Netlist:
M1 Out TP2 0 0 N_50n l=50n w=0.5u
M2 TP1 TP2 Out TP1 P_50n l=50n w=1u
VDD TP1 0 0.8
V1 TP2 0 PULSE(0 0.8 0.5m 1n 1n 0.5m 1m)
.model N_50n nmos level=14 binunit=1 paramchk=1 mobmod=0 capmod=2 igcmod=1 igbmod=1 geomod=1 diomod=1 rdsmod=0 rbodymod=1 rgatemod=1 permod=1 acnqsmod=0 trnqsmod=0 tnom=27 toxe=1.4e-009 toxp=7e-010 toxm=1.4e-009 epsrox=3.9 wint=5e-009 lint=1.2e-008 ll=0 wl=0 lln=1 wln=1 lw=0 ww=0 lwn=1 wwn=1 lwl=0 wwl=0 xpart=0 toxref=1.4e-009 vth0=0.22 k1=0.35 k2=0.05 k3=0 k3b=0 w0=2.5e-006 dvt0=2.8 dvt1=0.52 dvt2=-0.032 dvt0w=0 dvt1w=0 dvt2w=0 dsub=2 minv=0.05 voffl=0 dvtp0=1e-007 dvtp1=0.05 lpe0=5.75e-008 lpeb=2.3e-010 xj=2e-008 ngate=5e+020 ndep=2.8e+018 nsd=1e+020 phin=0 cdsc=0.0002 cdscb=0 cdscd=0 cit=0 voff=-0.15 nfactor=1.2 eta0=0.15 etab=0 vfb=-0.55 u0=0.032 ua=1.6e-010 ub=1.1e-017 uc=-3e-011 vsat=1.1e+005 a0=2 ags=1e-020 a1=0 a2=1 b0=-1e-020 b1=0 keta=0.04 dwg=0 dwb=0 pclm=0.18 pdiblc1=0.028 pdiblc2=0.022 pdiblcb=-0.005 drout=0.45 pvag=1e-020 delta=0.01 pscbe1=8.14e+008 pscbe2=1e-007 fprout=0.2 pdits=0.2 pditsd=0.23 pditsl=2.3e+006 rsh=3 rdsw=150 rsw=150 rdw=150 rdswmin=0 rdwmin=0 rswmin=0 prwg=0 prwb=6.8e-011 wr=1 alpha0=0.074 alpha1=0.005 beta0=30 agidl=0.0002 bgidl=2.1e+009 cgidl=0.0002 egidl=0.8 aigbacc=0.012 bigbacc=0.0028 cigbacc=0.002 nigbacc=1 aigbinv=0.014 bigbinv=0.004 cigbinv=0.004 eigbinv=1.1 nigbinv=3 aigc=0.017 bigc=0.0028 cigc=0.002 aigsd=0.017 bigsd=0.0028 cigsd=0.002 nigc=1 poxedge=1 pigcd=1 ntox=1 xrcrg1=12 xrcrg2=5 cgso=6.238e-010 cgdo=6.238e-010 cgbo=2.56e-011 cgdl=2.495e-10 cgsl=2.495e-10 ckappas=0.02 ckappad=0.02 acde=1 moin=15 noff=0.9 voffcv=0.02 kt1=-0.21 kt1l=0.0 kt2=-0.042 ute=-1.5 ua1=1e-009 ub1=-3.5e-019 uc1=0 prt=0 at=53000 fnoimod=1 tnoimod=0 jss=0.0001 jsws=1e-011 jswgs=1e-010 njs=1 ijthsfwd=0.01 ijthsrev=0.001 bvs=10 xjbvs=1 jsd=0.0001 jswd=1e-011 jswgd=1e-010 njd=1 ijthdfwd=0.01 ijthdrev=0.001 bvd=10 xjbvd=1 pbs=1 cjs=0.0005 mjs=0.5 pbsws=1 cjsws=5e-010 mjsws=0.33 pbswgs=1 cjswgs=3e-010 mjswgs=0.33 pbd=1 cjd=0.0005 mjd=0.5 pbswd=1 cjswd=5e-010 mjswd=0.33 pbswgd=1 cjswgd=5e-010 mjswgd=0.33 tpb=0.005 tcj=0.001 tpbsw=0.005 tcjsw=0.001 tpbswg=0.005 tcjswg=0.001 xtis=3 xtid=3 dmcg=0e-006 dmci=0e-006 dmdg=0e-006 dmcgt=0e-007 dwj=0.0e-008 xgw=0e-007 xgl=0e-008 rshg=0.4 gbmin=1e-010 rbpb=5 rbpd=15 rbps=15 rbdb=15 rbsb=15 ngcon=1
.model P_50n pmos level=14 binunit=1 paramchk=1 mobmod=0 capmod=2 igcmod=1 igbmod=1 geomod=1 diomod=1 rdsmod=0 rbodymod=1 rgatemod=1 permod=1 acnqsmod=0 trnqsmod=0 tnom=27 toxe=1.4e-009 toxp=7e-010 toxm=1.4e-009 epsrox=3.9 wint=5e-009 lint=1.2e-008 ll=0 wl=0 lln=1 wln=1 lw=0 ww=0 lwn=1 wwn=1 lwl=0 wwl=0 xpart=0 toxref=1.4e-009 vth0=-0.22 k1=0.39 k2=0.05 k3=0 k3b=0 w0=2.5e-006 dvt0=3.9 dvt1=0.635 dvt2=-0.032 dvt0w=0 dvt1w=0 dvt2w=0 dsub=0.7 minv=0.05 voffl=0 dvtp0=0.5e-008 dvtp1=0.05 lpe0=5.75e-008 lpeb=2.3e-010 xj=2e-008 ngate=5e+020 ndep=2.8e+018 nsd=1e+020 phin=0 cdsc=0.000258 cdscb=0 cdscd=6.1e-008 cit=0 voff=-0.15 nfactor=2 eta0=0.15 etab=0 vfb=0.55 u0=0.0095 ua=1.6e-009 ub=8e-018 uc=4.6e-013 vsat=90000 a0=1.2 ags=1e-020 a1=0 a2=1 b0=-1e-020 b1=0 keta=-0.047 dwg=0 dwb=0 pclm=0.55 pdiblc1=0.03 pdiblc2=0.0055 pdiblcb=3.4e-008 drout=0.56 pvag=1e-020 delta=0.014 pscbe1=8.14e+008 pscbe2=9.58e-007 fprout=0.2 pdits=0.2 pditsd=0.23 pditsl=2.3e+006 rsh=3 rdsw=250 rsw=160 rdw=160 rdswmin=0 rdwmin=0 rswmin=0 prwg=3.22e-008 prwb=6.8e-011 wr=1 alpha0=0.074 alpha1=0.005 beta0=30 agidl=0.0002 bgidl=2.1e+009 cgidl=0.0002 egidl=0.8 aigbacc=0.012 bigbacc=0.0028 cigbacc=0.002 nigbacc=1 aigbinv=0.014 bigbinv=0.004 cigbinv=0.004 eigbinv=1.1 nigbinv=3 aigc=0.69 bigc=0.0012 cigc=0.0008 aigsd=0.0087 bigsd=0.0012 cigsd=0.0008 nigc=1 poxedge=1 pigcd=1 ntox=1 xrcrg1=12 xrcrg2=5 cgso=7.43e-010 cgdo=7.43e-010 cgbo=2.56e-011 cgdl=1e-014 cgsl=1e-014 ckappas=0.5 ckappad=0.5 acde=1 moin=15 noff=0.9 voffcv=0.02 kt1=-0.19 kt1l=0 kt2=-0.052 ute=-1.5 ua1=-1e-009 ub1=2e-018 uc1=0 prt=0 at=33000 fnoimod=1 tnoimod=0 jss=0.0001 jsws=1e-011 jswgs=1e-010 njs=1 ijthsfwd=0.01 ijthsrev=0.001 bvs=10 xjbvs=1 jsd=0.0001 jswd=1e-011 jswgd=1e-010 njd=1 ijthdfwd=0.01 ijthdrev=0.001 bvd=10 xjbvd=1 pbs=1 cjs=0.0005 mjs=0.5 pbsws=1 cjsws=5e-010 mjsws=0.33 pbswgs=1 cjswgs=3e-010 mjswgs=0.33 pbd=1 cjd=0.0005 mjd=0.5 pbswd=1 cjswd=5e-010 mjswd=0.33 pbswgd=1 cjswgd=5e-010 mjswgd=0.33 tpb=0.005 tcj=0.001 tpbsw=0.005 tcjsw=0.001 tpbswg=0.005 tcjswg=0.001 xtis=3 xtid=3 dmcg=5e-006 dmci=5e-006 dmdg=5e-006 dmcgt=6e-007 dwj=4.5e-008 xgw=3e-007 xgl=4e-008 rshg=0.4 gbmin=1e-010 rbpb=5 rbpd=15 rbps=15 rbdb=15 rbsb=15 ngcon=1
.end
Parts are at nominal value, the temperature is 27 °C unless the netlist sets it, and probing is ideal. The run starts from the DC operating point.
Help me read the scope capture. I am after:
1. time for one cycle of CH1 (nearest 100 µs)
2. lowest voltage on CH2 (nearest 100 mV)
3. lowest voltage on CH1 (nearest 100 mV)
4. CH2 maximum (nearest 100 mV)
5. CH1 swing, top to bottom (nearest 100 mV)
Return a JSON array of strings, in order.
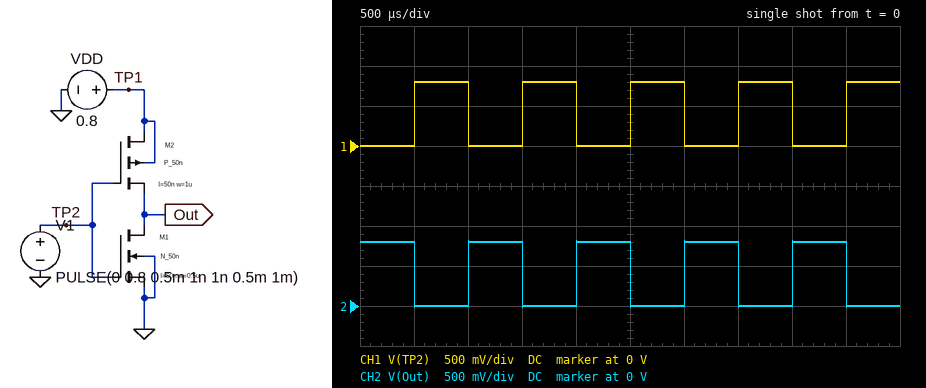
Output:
["1.0 ms", "0 V", "0 V", "800 mV", "800 mV"]
